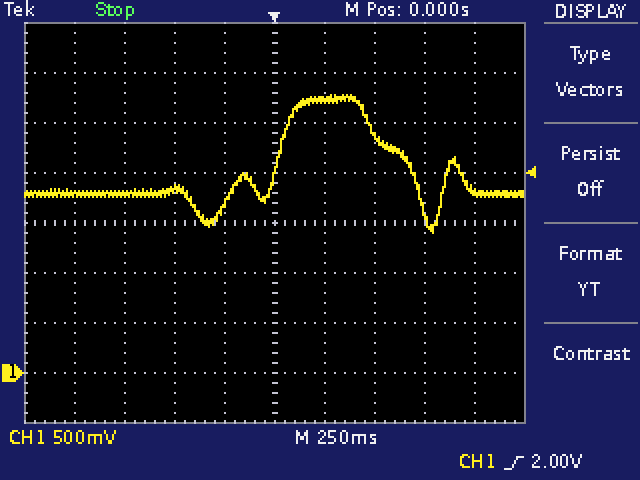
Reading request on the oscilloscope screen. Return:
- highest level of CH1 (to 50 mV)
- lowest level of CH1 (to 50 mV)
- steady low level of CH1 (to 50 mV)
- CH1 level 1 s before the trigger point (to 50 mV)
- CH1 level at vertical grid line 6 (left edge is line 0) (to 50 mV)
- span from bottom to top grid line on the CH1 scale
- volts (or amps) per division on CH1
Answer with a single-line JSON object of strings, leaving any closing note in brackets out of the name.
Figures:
{"highest level of CH1": "2.80 V", "lowest level of CH1": "1.40 V", "steady low level of CH1": "1.80 V", "CH1 level 1 s before the trigger point": "1.80 V", "CH1 level at vertical grid line 6 (left edge is line 0)": "2.75 V", "span from bottom to top grid line on the CH1 scale": "4 V", "volts (or amps) per division on CH1": "500 mV"}
